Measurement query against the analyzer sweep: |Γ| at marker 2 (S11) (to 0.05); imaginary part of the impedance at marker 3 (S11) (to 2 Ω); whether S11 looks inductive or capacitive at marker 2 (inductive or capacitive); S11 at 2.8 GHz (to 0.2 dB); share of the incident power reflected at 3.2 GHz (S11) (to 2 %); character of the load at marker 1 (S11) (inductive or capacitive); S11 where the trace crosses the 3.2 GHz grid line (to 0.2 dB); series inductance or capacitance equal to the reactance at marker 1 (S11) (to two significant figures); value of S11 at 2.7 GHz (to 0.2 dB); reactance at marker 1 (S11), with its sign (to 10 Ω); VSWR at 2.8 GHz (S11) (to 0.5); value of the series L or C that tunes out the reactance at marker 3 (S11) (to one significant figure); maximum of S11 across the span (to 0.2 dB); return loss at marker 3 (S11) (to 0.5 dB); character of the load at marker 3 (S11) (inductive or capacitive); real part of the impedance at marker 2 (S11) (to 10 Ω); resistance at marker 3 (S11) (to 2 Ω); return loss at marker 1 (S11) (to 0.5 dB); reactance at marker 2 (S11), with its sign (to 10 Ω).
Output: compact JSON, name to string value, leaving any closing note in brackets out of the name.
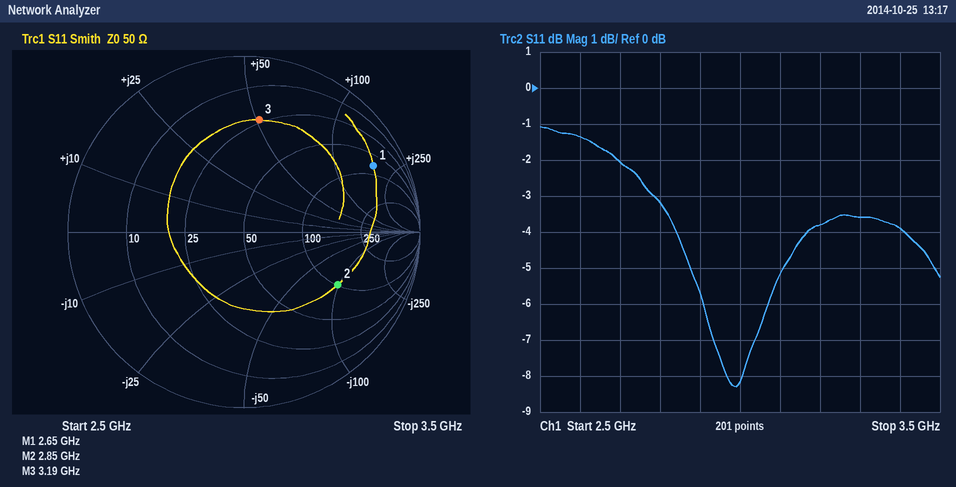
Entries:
{"|Γ| at marker 2 (S11)": "0.60", "imaginary part of the impedance at marker 3 (S11)": "+52 Ω", "whether S11 looks inductive or capacitive at marker 2": "capacitive", "S11 at 2.8 GHz": "-3.2 dB", "share of the incident power reflected at 3.2 GHz (S11)": "42 %", "character of the load at marker 1 (S11)": "inductive", "S11 where the trace crosses the 3.2 GHz grid line": "-3.8 dB", "series inductance or capacitance equal to the reactance at marker 1 (S11)": "11 nH", "value of S11 at 2.7 GHz": "-2.0 dB", "reactance at marker 1 (S11), with its sign": "+180 Ω", "VSWR at 2.8 GHz (S11)": "5.5", "value of the series L or C that tunes out the reactance at marker 3 (S11)": "1.0 pF", "maximum of S11 across the span": "-1.0 dB", "return loss at marker 3 (S11)": "4.0 dB", "character of the load at marker 3 (S11)": "inductive", "real part of the impedance at marker 2 (S11)": "100 Ω", "resistance at marker 3 (S11)": "24 Ω", "return loss at marker 1 (S11)": "1.5 dB", "reactance at marker 2 (S11), with its sign": "-100 Ω"}
